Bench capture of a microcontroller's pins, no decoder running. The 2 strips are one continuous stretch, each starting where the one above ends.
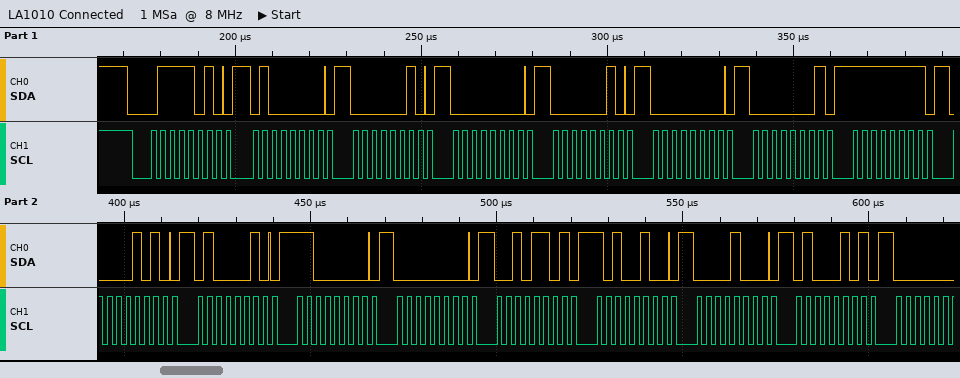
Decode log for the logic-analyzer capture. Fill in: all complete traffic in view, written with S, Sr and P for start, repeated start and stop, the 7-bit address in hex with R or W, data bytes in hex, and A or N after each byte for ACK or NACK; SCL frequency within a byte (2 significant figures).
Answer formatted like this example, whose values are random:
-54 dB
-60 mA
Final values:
S 3DW A 40 A 02 A 00 A 02 A 00 A 01 A FF A 0A A 42 A C0 A 00 A 2D A A4 A 08 A 45 A
400 kHz
